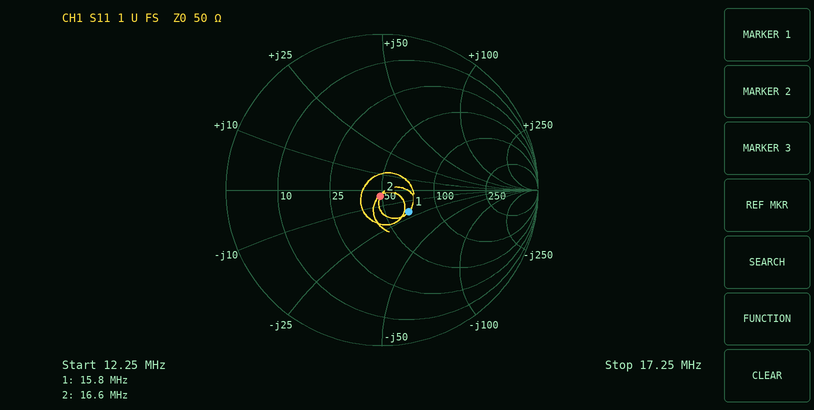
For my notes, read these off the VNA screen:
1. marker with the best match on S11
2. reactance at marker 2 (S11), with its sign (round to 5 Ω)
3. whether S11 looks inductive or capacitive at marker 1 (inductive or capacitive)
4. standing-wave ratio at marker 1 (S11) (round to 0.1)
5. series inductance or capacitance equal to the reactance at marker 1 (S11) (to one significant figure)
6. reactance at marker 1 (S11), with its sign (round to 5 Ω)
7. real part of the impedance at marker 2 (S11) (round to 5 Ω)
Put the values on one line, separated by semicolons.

marker 2; -5 Ω; capacitive; 1.6; 500 pF; -20 Ω; 50 Ω
